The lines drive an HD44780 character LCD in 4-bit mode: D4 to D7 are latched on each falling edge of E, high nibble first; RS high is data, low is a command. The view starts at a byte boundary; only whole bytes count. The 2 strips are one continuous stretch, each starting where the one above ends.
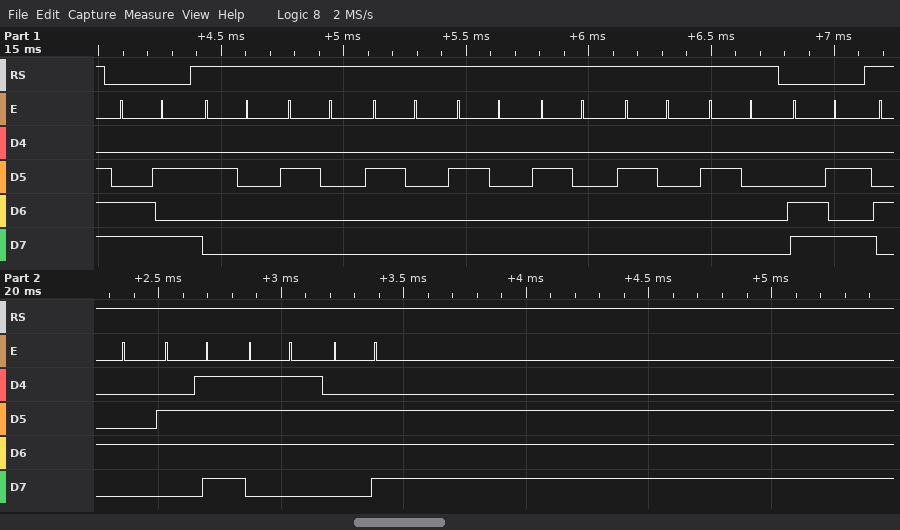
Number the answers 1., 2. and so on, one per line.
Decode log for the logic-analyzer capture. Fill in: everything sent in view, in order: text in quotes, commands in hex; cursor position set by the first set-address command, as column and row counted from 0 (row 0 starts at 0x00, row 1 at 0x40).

1. 0xCA "       " 0xCA "Down"
2. column 10, row 1
